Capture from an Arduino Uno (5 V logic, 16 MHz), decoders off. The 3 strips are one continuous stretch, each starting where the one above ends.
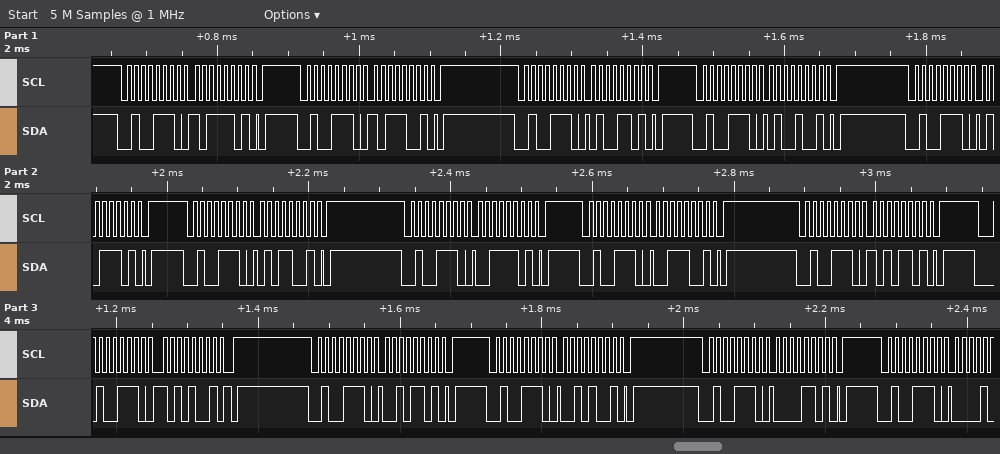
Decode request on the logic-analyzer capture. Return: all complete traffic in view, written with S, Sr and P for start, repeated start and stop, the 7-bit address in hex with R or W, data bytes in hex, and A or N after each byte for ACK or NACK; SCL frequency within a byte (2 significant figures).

S 27W A BD A P S 27W A B9 A P S 27W A 4D A P S 27W A 49 A P S 27W A 5D A P S 27W A 59 A P S 27W A 3D A P S 27W A 39 A P S 27W A AD A P S 27W A A9 A P S 27W A 2D A P S 27W A 29 A P S 27W A 0D A P S 27W A
100 kHz
